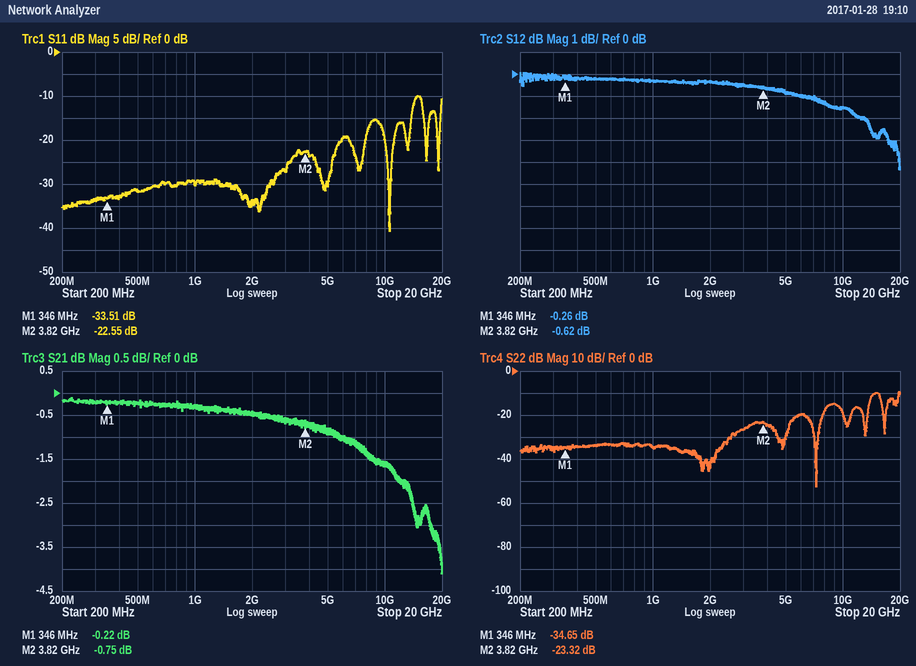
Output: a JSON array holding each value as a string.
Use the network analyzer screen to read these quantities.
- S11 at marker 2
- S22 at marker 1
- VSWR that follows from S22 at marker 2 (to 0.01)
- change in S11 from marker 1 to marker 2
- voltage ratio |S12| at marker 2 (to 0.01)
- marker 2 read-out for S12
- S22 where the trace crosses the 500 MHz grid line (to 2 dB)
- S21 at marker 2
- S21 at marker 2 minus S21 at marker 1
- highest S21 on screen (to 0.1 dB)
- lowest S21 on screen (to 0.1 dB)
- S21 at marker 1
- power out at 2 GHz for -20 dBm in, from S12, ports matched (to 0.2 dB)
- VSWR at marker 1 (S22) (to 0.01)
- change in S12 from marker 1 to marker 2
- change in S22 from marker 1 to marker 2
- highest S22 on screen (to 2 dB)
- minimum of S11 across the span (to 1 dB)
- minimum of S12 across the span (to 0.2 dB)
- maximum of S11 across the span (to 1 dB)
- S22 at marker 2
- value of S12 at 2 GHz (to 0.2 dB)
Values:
["-22.55 dB", "-34.65 dB", "1.15", "10.96 dB", "0.93", "-0.62 dB", "-34 dB", "-0.75 dB", "-0.53 dB", "-0.1 dB", "-4.1 dB", "-0.22 dB", "-20.4 dBm", "1.04", "-0.36 dB", "11.33 dB", "-10 dB", "-41 dB", "-4.4 dB", "-10 dB", "-23.32 dB", "-0.4 dB"]
